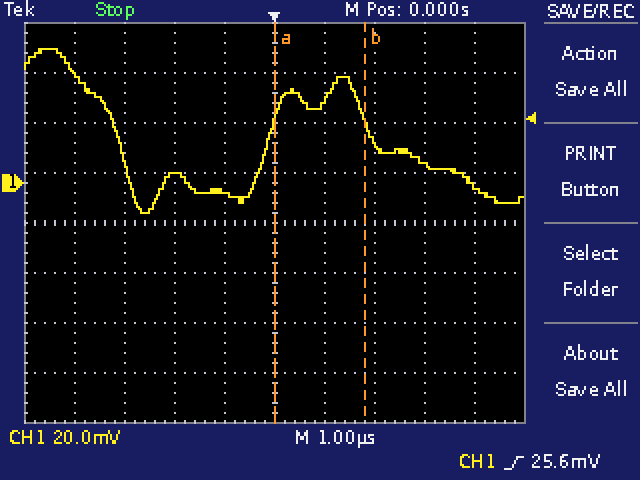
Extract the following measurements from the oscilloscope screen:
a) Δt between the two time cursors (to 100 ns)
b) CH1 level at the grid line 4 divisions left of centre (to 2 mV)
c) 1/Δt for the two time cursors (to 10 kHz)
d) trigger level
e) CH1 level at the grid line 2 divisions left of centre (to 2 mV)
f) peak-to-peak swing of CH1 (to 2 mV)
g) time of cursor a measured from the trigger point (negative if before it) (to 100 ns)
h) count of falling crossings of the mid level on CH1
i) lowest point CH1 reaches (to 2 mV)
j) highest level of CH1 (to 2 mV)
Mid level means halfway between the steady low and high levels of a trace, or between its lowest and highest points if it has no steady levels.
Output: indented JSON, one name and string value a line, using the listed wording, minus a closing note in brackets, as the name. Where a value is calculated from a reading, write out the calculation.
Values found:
{
  "Δt between the two time cursors": "1.8 µs",
  "CH1 level at the grid line 4 divisions left of centre": "44 mV",
  "1/Δt for the two time cursors": "1 / 1.8 µs ≈ 560 kHz",
  "trigger level": "25.6 mV",
  "CH1 level at the grid line 2 divisions left of centre": "4 mV",
  "peak-to-peak swing of CH1": "54 mV − (-12 mV) = 66 mV",
  "time of cursor a measured from the trigger point (negative if before it)": "0.0 µs",
  "count of falling crossings of the mid level on CH1": "2",
  "lowest point CH1 reaches": "-12 mV",
  "highest level of CH1": "54 mV"
}
